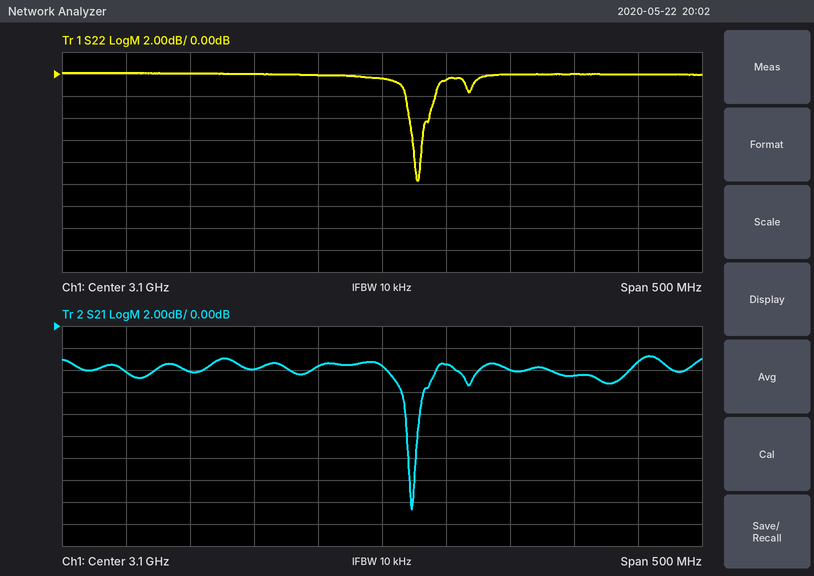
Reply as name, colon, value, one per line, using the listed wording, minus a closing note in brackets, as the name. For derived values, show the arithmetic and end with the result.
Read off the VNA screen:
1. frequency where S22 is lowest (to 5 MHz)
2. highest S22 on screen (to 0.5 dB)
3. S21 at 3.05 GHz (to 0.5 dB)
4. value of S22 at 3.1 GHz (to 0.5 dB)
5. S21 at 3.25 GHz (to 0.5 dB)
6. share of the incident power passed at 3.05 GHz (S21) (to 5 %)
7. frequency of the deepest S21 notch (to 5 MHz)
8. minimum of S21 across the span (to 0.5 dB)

frequency where S22 is lowest: 3.130 GHz
highest S22 on screen: 0.0 dB
S21 at 3.05 GHz: -3.5 dB
value of S22 at 3.1 GHz: -0.5 dB
S21 at 3.25 GHz: -4.5 dB
share of the incident power passed at 3.05 GHz (S21): 10^(-3.5/10) ≈ 45 %
frequency of the deepest S21 notch: 3.125 GHz
minimum of S21 across the span: -16.5 dB
